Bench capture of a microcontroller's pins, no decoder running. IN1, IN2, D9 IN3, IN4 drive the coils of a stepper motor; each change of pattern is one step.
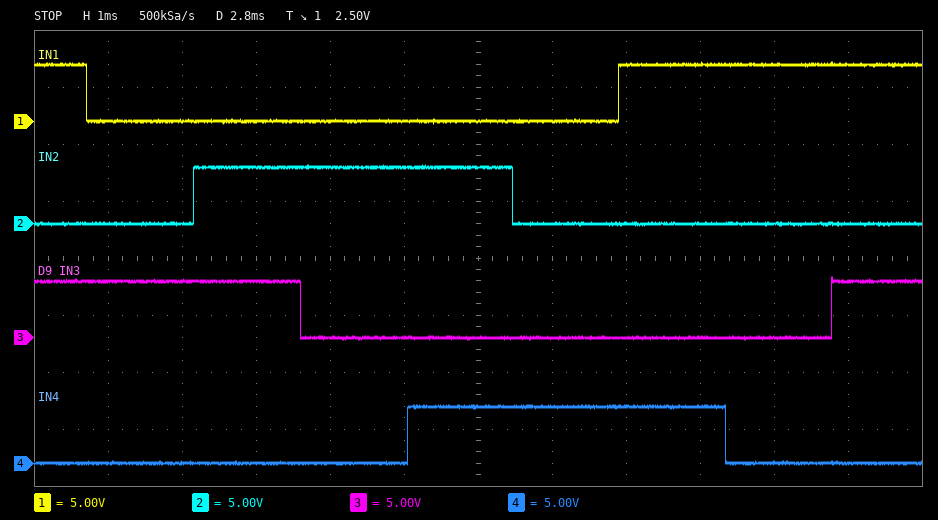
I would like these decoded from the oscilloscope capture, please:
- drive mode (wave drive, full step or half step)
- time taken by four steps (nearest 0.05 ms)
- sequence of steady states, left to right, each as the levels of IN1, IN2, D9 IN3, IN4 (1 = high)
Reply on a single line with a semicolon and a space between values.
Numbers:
half step; 5.75 ms; 1010 0010 0110 0100 0101 0001 1001 1000 1010
